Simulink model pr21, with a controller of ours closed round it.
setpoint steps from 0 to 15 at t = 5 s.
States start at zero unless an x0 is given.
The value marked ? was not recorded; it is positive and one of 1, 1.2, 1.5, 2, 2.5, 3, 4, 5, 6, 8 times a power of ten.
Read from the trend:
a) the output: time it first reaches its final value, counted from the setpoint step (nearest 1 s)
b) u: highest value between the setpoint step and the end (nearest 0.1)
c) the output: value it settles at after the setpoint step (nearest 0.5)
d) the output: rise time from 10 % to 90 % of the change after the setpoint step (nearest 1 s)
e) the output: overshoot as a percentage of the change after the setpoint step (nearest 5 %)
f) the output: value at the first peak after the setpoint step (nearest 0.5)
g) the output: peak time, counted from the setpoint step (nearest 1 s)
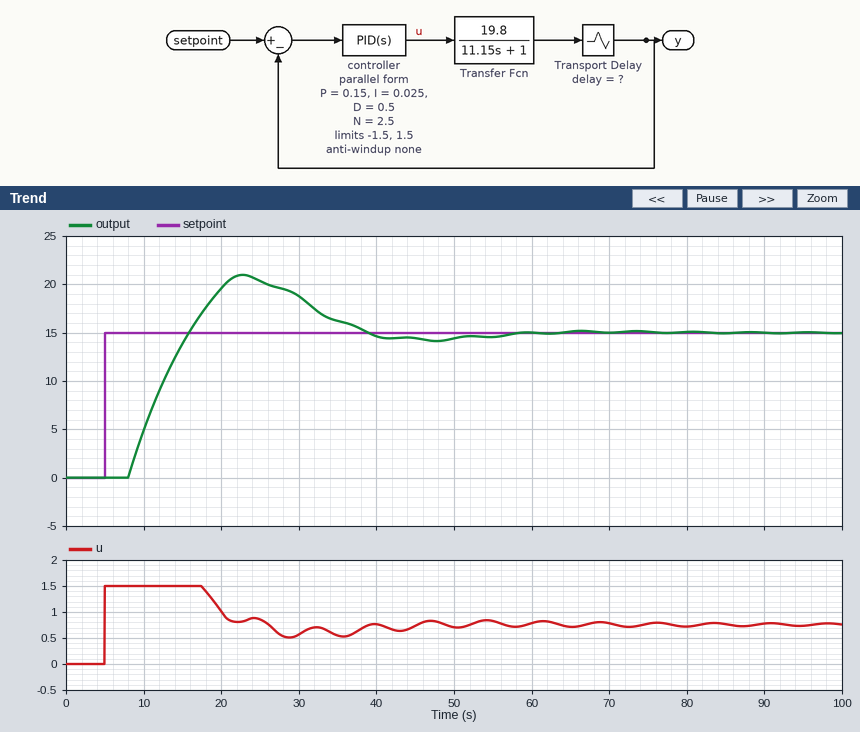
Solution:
11 s
1.5
15.0
6 s
40 %
21.0
18 s
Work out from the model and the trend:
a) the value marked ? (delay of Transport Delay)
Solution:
3
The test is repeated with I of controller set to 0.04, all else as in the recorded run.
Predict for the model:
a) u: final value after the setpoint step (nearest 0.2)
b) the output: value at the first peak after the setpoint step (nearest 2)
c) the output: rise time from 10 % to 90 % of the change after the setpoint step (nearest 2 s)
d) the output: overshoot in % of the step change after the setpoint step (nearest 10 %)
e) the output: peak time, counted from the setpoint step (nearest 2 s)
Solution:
0.8
24
6 s
60 %
22 s
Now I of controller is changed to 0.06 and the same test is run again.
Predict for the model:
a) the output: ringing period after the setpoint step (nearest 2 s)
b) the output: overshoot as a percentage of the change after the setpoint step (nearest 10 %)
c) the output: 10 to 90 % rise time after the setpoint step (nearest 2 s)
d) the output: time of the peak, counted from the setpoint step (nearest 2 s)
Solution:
24 s
70 %
6 s
24 s
